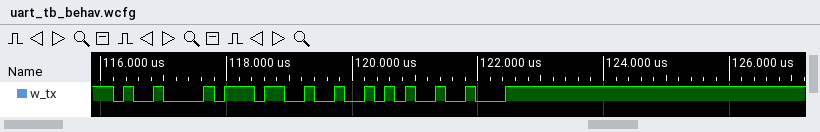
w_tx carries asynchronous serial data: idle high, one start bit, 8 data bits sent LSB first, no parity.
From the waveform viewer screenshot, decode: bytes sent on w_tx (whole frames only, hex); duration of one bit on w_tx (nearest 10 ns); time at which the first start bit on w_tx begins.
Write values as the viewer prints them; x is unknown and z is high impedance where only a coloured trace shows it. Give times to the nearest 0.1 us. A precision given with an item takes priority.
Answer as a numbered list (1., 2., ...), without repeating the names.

1. 09, 37, 52, 12
2. 160 ns
3. 116.2 us
